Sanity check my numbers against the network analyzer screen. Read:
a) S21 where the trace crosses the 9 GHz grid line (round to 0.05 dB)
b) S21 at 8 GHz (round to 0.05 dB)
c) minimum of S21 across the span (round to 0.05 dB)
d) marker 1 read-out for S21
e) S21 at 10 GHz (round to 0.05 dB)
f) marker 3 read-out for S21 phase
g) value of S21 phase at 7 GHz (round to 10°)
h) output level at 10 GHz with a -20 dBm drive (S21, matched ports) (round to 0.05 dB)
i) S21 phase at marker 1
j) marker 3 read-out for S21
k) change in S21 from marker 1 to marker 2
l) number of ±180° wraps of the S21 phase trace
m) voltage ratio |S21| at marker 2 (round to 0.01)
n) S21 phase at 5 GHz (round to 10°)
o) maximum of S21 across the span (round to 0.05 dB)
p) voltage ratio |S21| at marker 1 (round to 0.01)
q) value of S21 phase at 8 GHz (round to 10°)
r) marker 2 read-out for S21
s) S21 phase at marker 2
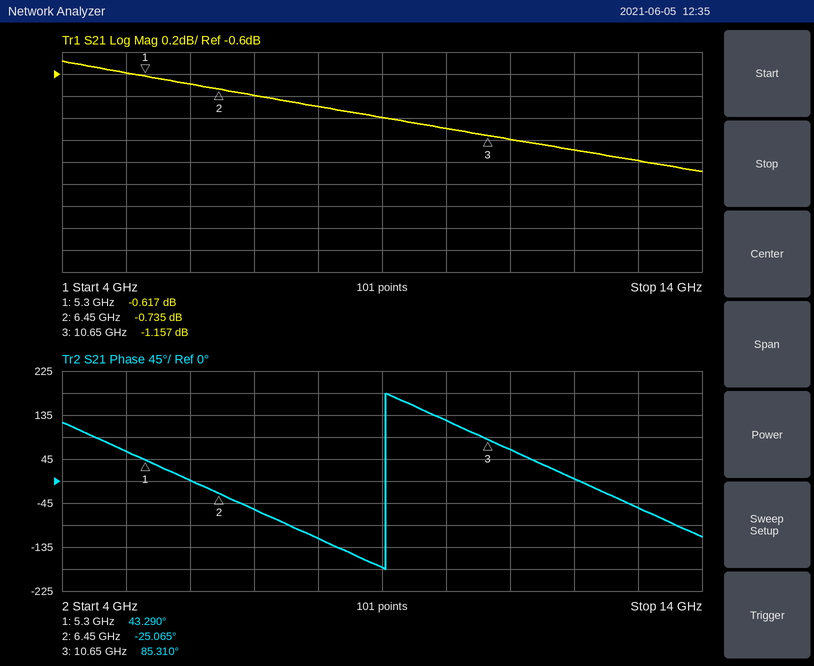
-1.00 dB
-0.90 dB
-1.50 dB
-0.617 dB
-1.10 dB
85.310°
-60°
-21.10 dBm
43.290°
-1.157 dB
-0.118 dB
1
0.92
60°
-0.50 dB
0.93
-120°
-0.735 dB
-25.065°
